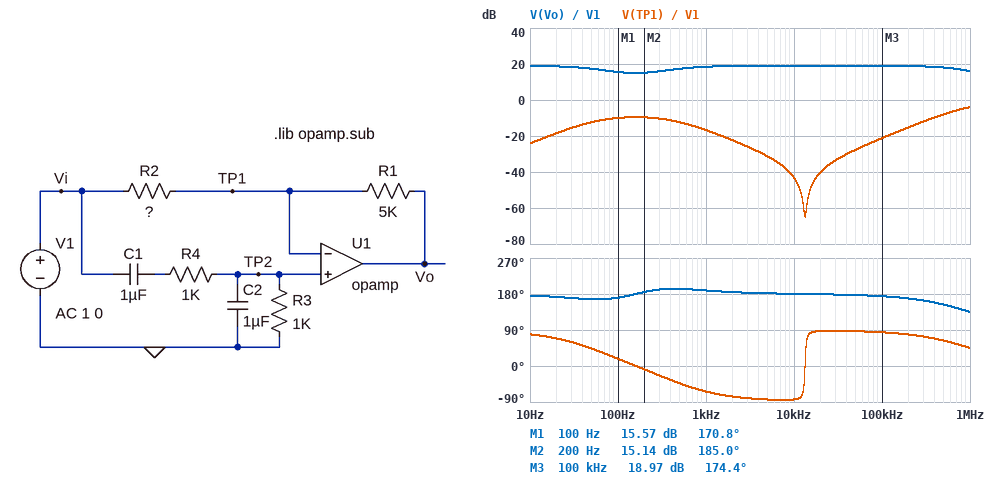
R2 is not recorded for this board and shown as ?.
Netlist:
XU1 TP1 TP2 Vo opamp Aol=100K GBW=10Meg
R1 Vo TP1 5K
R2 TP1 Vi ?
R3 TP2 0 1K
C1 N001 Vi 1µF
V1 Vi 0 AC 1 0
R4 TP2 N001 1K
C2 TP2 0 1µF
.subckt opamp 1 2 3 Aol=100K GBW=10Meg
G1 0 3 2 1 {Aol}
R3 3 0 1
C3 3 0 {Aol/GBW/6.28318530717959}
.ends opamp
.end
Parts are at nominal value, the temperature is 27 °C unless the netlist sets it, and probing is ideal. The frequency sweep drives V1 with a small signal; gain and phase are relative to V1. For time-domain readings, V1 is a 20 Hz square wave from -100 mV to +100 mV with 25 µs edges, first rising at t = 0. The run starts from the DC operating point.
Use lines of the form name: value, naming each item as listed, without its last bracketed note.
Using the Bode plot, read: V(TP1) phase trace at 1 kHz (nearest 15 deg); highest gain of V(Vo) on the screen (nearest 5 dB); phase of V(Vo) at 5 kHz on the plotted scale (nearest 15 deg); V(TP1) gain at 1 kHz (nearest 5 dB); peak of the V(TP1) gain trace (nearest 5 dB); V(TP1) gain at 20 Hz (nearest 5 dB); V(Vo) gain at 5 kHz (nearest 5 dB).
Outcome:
V(TP1) phase trace at 1 kHz: -60 deg
highest gain of V(Vo) on the screen: 20 dB
phase of V(Vo) at 5 kHz on the plotted scale: 180 deg
V(TP1) gain at 1 kHz: -15 dB
peak of the V(TP1) gain trace: -5 dB
V(TP1) gain at 20 Hz: -20 dB
V(Vo) gain at 5 kHz: 20 dB
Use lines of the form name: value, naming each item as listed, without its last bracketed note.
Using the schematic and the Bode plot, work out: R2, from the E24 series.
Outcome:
R2, from the E24 series: 560 Ω
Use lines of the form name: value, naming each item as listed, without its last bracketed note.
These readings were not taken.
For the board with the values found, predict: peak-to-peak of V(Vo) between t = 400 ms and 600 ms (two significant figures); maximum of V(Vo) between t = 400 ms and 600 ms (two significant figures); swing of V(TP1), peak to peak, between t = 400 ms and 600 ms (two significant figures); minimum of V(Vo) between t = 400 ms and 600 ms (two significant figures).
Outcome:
peak-to-peak of V(Vo) between t = 400 ms and 600 ms: 1.8 V
maximum of V(Vo) between t = 400 ms and 600 ms: 890 mV
swing of V(TP1), peak to peak, between t = 400 ms and 600 ms: 110 mV
minimum of V(Vo) between t = 400 ms and 600 ms: -890 mV
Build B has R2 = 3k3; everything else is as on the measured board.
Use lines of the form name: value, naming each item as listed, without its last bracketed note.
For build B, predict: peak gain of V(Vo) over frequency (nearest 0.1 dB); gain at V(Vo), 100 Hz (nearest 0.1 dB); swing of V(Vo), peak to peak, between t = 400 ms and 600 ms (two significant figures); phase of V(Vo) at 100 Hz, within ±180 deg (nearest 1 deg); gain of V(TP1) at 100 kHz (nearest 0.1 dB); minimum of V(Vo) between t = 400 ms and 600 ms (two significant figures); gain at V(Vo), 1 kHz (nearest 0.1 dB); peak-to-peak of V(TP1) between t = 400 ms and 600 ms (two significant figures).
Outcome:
peak gain of V(Vo) over frequency: 3.6 dB
gain at V(Vo), 100 Hz: -2.0 dB
swing of V(Vo), peak to peak, between t = 400 ms and 600 ms: 300 mV
phase of V(Vo) at 100 Hz, within ±180 deg: 162 deg
gain of V(TP1) at 100 kHz: -37.4 dB
minimum of V(Vo) between t = 400 ms and 600 ms: -150 mV
gain at V(Vo), 1 kHz: 2.9 dB
peak-to-peak of V(TP1) between t = 400 ms and 600 ms: 110 mV
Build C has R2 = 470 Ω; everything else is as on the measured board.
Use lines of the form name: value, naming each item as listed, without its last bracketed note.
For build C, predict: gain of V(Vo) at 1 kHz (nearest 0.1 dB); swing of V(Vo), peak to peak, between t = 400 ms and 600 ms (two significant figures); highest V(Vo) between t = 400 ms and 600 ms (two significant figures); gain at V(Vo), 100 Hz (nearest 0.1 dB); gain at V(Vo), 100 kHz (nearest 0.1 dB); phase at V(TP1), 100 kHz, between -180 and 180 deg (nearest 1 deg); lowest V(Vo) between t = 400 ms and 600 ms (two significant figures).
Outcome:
gain of V(Vo) at 1 kHz: 20.0 dB
swing of V(Vo), peak to peak, between t = 400 ms and 600 ms: 2.1 V
highest V(Vo) between t = 400 ms and 600 ms: 1.1 V
gain at V(Vo), 100 Hz: 17.2 dB
gain at V(Vo), 100 kHz: 20.5 dB
phase at V(TP1), 100 kHz, between -180 and 180 deg: 83 deg
lowest V(Vo) between t = 400 ms and 600 ms: -1.1 V
